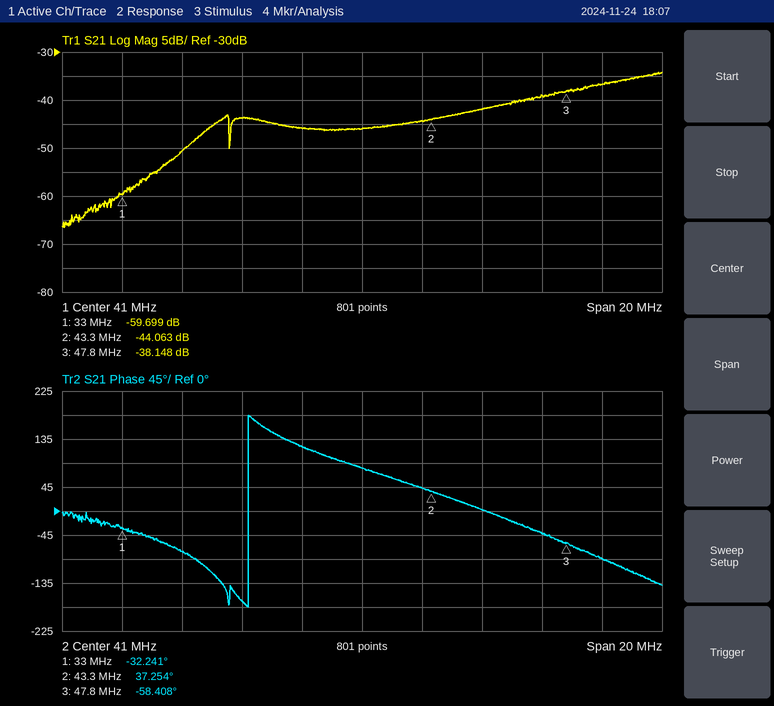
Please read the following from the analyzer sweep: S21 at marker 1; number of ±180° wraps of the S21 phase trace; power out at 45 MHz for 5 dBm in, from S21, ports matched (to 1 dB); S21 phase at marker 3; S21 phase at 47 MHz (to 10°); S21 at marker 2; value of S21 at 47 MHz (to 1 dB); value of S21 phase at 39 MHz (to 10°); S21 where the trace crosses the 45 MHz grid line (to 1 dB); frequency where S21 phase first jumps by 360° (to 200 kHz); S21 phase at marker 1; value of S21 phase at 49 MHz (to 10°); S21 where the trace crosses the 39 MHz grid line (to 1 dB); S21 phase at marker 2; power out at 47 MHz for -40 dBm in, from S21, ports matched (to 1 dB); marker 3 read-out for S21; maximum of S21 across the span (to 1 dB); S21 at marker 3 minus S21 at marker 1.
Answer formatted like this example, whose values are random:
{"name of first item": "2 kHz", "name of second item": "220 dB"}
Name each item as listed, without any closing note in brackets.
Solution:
{"S21 at marker 1": "-59.699 dB", "number of ±180° wraps of the S21 phase trace": "1", "power out at 45 MHz for 5 dBm in, from S21, ports matched": "-37 dBm", "S21 phase at marker 3": "-58.408°", "S21 phase at 47 MHz": "-40°", "S21 at marker 2": "-44.063 dB", "value of S21 at 47 MHz": "-39 dB", "value of S21 phase at 39 MHz": "120°", "S21 where the trace crosses the 45 MHz grid line": "-42 dB", "frequency where S21 phase first jumps by 360°": "37.2 MHz", "S21 phase at marker 1": "-32.241°", "value of S21 phase at 49 MHz": "-90°", "S21 where the trace crosses the 39 MHz grid line": "-46 dB", "S21 phase at marker 2": "37.254°", "power out at 47 MHz for -40 dBm in, from S21, ports matched": "-79 dBm", "marker 3 read-out for S21": "-38.148 dB", "maximum of S21 across the span": "-34 dB", "S21 at marker 3 minus S21 at marker 1": "21.551 dB"}
